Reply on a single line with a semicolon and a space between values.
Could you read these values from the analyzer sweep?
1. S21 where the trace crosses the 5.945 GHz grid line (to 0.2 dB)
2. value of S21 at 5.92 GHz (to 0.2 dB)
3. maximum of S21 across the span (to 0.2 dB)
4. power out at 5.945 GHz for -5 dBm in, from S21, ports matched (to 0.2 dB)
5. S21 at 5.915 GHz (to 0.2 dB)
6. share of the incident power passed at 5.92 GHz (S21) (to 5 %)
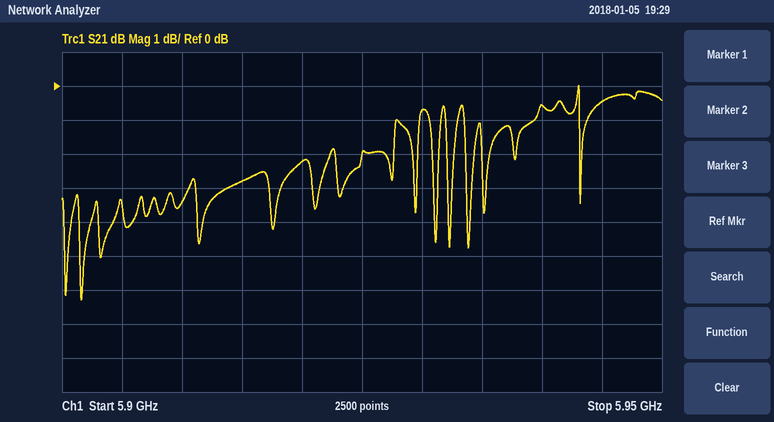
-0.4 dB; -2.2 dB; 0.0 dB; -5.4 dBm; -2.8 dB; 60 %
